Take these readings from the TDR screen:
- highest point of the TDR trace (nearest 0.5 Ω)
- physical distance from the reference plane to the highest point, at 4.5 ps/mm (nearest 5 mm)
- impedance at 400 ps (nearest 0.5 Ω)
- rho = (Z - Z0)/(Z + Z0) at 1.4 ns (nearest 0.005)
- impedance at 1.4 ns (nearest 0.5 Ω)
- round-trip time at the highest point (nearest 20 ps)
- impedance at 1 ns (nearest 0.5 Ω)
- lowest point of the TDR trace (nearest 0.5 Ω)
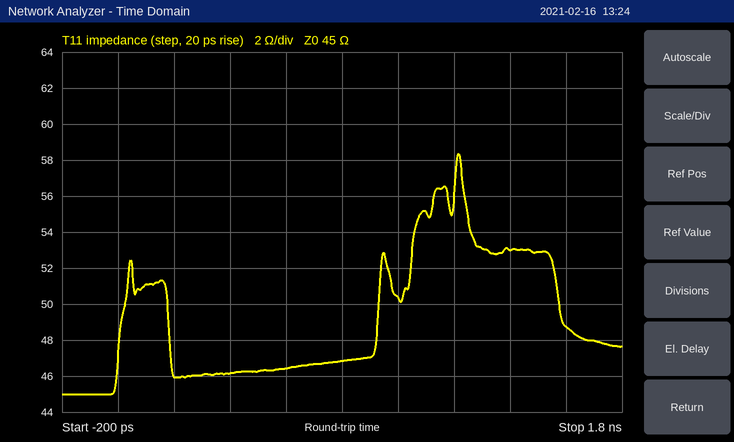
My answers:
58.5 Ω
135 mm
46.0 Ω
+0.080
53.0 Ω
1.22 ns
50.5 Ω
45.0 Ω
